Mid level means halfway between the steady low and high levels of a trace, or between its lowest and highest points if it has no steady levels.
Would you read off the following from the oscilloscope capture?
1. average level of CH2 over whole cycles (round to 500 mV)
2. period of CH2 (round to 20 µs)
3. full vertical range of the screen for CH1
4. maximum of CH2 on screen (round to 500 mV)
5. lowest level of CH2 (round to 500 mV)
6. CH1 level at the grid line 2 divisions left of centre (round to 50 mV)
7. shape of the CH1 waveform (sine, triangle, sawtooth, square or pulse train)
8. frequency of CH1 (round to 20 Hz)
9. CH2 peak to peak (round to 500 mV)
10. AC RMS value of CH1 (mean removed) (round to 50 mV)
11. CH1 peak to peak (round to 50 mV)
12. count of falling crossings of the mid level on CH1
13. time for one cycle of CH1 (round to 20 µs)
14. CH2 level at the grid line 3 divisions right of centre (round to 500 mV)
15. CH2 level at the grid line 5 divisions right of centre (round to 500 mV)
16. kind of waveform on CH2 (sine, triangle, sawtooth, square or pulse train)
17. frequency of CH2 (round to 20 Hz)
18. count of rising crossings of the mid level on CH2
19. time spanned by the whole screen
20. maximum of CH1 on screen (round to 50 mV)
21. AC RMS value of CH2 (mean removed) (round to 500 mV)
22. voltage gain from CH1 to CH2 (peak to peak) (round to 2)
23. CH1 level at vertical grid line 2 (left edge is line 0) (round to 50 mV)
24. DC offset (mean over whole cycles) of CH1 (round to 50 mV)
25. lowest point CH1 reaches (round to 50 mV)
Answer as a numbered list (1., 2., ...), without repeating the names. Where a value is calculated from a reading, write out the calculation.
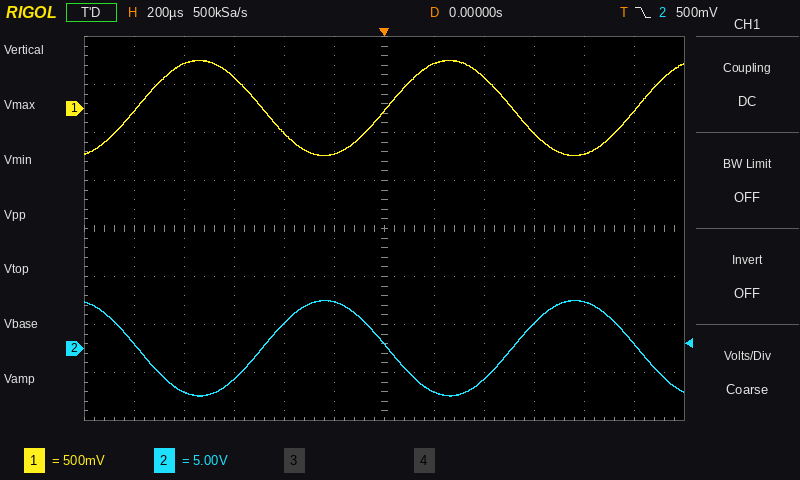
1. (5.0 V + (-5.0 V)) / 2 ≈ 0.0 V
2. 1.00 ms
3. 4 V
4. 5.0 V
5. -5.0 V
6. -250 mV
7. sine
8. 1 / 1.00 ms ≈ 1.00 kHz
9. 5.0 V − (-5.0 V) = 10.0 V
10. 1.00 V / (2√2) ≈ 354 mV, so 350 mV to the nearest 50 mV
11. 500 mV − (-500 mV) = 1.00 V
12. 2
13. 1.00 ms
14. 2.5 V
15. 500 mV
16. sine
17. 1 / 1.00 ms ≈ 1.00 kHz
18. 2
19. 2.4 ms
20. 500 mV
21. 10.0 V / (2√2) ≈ 3.5 V
22. 10.0 V / 1.00 V ≈ 10
23. 450 mV
24. (500 mV + (-500 mV)) / 2 ≈ 0 mV
25. -500 mV
